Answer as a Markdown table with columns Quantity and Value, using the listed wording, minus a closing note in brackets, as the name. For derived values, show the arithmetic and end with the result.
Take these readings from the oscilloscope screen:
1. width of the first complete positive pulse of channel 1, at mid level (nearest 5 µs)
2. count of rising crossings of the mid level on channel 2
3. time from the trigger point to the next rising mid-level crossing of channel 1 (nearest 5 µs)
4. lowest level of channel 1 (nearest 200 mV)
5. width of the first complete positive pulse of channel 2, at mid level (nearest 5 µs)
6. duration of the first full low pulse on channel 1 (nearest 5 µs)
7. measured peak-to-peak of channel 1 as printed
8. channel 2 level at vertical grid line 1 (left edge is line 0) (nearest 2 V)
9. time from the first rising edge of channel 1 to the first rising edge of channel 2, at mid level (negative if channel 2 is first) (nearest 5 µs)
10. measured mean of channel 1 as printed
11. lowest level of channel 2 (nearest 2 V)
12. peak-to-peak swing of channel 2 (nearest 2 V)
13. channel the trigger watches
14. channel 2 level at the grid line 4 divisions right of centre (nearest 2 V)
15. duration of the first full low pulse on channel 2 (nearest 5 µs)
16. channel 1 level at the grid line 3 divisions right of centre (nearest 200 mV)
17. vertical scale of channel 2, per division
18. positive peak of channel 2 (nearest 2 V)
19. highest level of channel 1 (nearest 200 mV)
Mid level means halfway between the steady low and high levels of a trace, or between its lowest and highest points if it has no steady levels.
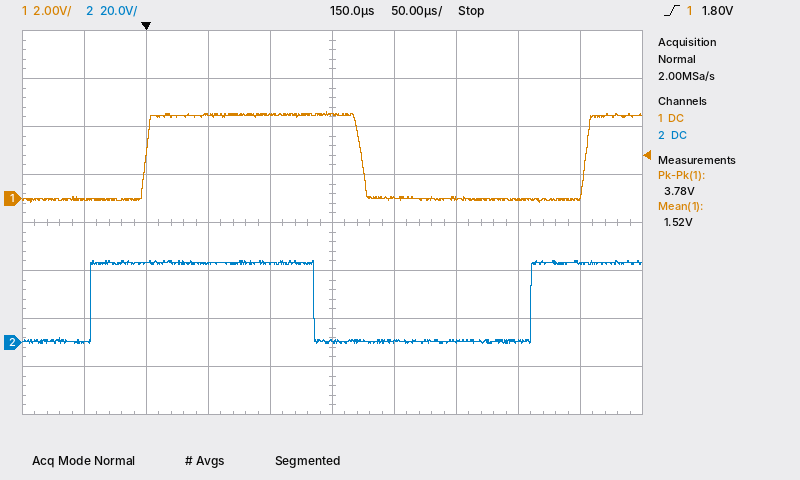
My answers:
| Quantity | Value |
|---|---|
| width of the first complete positive pulse of channel 1, at mid level | 175 µs |
| count of rising crossings of the mid level on channel 2 | 2 |
| time from the trigger point to the next rising mid-level crossing of channel 1 | 355 µs |
| lowest level of channel 1 | -200 mV |
| width of the first complete positive pulse of channel 2, at mid level | 180 µs |
| duration of the first full low pulse on channel 1 | 180 µs |
| measured peak-to-peak of channel 1 as printed | 3.78 V |
| channel 2 level at vertical grid line 1 (left edge is line 0) | 0 V |
| time from the first rising edge of channel 1 to the first rising edge of channel 2, at mid level (negative if channel 2 is first) | -45 µs |
| measured mean of channel 1 as printed | 1.52 V |
| lowest level of channel 2 | 0 V |
| peak-to-peak swing of channel 2 | 34 V − (0 V) = 34 V |
| channel the trigger watches | channel 1 |
| channel 2 level at the grid line 4 divisions right of centre | 34 V |
| duration of the first full low pulse on channel 2 | 175 µs |
| channel 1 level at the grid line 3 divisions right of centre | 0.0 V |
| vertical scale of channel 2, per division | 20 V |
| positive peak of channel 2 | 34 V |
| highest level of channel 1 | 3.6 V |
